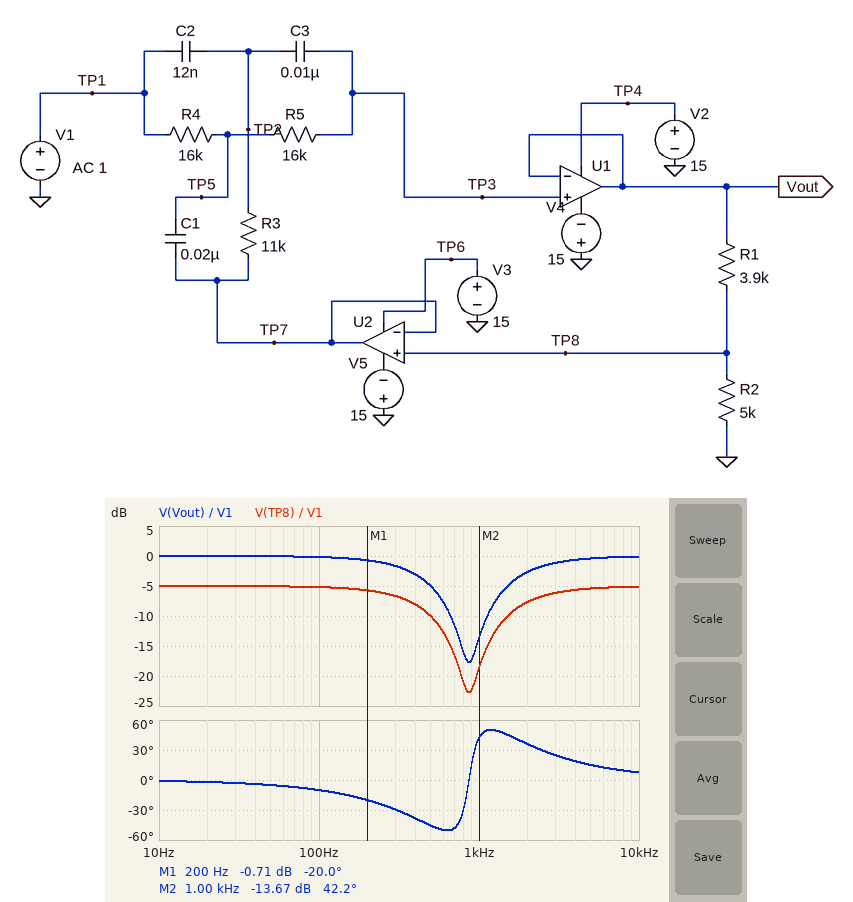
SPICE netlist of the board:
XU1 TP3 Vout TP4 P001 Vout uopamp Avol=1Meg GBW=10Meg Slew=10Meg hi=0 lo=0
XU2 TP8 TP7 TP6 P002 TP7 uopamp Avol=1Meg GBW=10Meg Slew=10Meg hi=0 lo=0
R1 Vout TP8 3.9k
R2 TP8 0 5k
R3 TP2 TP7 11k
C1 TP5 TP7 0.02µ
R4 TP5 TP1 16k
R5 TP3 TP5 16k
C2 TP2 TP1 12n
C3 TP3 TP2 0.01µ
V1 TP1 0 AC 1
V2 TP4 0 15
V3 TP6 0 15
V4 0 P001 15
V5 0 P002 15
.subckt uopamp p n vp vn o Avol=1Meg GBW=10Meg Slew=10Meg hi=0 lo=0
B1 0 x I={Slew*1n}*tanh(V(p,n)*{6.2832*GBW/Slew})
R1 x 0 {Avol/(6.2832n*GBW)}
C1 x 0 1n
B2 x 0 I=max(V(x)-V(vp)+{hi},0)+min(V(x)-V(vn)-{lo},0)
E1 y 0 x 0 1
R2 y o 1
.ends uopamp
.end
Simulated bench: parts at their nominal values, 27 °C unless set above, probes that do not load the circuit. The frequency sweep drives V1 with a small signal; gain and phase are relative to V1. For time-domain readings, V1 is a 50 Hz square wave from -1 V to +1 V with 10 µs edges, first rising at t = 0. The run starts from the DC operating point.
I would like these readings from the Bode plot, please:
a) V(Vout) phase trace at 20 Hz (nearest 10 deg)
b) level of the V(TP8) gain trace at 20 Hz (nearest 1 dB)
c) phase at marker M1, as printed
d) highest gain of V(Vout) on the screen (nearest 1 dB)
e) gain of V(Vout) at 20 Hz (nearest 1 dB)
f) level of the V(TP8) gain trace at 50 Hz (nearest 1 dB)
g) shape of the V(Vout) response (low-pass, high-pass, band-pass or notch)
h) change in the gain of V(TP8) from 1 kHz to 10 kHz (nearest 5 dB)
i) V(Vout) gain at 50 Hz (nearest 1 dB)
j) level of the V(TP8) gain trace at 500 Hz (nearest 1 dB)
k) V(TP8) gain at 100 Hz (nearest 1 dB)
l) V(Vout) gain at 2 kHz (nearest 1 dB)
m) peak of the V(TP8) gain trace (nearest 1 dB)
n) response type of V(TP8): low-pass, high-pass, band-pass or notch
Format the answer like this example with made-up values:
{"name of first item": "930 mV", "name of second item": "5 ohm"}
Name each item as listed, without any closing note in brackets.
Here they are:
{"V(Vout) phase trace at 20 Hz": "0 deg", "level of the V(TP8) gain trace at 20 Hz": "-5 dB", "phase at marker M1, as printed": "-20.0 deg", "highest gain of V(Vout) on the screen": "0 dB", "gain of V(Vout) at 20 Hz": "0 dB", "level of the V(TP8) gain trace at 50 Hz": "-5 dB", "shape of the V(Vout) response": "notch", "change in the gain of V(TP8) from 1 kHz to 10 kHz": "15 dB", "V(Vout) gain at 50 Hz": "0 dB", "level of the V(TP8) gain trace at 500 Hz": "-10 dB", "V(TP8) gain at 100 Hz": "-5 dB", "V(Vout) gain at 2 kHz": "-3 dB", "peak of the V(TP8) gain trace": "-5 dB", "response type of V(TP8): low-pass, high-pass, band-pass or notch": "notch"}
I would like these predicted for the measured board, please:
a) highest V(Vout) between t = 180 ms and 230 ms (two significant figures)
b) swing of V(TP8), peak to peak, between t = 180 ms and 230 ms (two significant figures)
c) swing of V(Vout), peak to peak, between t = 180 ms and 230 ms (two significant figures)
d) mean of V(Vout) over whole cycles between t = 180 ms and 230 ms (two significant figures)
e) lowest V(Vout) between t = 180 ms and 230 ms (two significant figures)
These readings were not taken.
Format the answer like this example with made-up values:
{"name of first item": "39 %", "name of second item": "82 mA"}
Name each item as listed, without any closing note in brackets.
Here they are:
{"highest V(Vout) between t = 180 ms and 230 ms": "1.0 V", "swing of V(TP8), peak to peak, between t = 180 ms and 230 ms": "1.1 V", "swing of V(Vout), peak to peak, between t = 180 ms and 230 ms": "2.0 V", "mean of V(Vout) over whole cycles between t = 180 ms and 230 ms": "190 mV", "lowest V(Vout) between t = 180 ms and 230 ms": "-1.0 V"}
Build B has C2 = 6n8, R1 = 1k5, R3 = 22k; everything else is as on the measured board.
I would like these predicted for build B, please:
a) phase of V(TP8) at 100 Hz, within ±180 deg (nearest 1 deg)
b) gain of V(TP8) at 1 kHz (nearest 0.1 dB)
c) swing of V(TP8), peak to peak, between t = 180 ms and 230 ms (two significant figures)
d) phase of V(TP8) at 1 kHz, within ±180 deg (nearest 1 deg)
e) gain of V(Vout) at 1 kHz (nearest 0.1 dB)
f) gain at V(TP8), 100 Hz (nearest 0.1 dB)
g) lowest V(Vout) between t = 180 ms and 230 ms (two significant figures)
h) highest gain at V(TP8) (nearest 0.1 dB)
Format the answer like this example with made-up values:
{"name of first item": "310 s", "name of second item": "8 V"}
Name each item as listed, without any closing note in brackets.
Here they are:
{"phase of V(TP8) at 100 Hz, within ±180 deg": "-5 deg", "gain of V(TP8) at 1 kHz": "-11.3 dB", "swing of V(TP8), peak to peak, between t = 180 ms and 230 ms": "1.6 V", "phase of V(TP8) at 1 kHz, within ±180 deg": "4 deg", "gain of V(Vout) at 1 kHz": "-9.0 dB", "gain at V(TP8), 100 Hz": "-2.4 dB", "lowest V(Vout) between t = 180 ms and 230 ms": "-1.0 V", "highest gain at V(TP8)": "-2.3 dB"}
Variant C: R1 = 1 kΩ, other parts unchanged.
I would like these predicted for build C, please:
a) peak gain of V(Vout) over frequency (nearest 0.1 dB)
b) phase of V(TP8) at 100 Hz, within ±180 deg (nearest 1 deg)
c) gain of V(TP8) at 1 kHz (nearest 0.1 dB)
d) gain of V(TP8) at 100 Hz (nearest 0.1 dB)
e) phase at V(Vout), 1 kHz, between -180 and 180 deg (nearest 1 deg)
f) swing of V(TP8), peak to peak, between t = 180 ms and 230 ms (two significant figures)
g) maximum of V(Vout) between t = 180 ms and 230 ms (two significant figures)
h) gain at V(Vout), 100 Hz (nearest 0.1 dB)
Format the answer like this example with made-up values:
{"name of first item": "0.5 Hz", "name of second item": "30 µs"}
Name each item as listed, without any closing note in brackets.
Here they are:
{"peak gain of V(Vout) over frequency": "0 dB", "phase of V(TP8) at 100 Hz, within ±180 deg": "-4 deg", "gain of V(TP8) at 1 kHz": "-8.9 dB", "gain of V(TP8) at 100 Hz": "-1.6 dB", "phase at V(Vout), 1 kHz, between -180 and 180 deg": "32 deg", "swing of V(TP8), peak to peak, between t = 180 ms and 230 ms": "2.0 V", "maximum of V(Vout) between t = 180 ms and 230 ms": "1.2 V", "gain at V(Vout), 100 Hz": "0 dB"}
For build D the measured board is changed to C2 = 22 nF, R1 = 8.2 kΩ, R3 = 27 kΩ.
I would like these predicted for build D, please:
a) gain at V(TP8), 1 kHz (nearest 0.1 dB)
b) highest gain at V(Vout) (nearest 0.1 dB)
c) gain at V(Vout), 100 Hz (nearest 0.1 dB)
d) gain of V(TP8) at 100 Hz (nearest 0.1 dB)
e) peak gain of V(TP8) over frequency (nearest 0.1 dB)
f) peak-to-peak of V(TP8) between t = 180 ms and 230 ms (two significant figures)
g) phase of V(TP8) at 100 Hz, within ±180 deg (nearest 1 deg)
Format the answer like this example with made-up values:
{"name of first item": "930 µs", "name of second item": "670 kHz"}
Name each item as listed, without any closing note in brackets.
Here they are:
{"gain at V(TP8), 1 kHz": "-15.0 dB", "highest gain at V(Vout)": "0 dB", "gain at V(Vout), 100 Hz": "-0.7 dB", "gain of V(TP8) at 100 Hz": "-9.1 dB", "peak gain of V(TP8) over frequency": "-8.4 dB", "peak-to-peak of V(TP8) between t = 180 ms and 230 ms": "760 mV", "phase of V(TP8) at 100 Hz, within ±180 deg": "-13 deg"}
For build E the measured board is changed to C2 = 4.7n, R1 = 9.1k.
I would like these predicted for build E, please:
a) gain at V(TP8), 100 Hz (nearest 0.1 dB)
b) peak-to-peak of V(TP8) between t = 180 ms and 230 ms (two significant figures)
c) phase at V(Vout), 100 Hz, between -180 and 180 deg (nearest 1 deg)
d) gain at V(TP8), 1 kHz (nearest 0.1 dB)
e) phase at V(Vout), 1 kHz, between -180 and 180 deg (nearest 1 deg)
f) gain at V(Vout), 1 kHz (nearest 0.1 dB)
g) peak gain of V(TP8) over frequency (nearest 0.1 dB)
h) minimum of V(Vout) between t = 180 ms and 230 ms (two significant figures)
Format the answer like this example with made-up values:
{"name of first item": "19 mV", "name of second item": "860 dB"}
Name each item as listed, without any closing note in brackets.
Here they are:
{"gain at V(TP8), 100 Hz": "-9.3 dB", "peak-to-peak of V(TP8) between t = 180 ms and 230 ms": "710 mV", "phase at V(Vout), 100 Hz, between -180 and 180 deg": "-15 deg", "gain at V(TP8), 1 kHz": "-26.5 dB", "phase at V(Vout), 1 kHz, between -180 and 180 deg": "-82 deg", "gain at V(Vout), 1 kHz": "-17.5 dB", "peak gain of V(TP8) over frequency": "-9.0 dB", "minimum of V(Vout) between t = 180 ms and 230 ms": "-1.0 V"}
